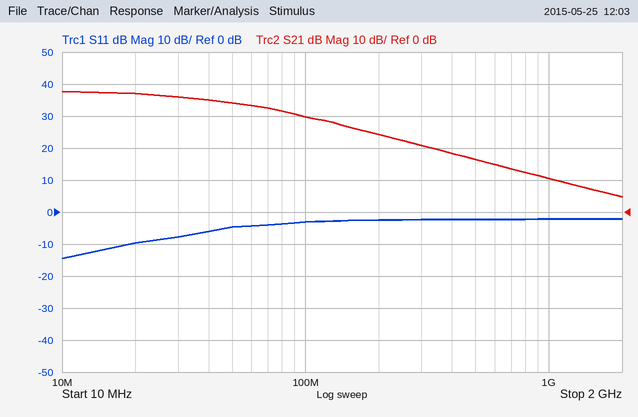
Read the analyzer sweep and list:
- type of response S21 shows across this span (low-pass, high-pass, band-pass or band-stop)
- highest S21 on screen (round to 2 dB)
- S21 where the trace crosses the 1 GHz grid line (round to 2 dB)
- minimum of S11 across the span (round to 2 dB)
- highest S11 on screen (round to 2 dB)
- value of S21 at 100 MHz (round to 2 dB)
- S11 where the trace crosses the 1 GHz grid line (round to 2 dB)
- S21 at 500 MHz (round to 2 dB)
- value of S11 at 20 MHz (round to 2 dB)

low-pass
38 dB
10 dB
-14 dB
-2 dB
30 dB
-2 dB
16 dB
-10 dB
